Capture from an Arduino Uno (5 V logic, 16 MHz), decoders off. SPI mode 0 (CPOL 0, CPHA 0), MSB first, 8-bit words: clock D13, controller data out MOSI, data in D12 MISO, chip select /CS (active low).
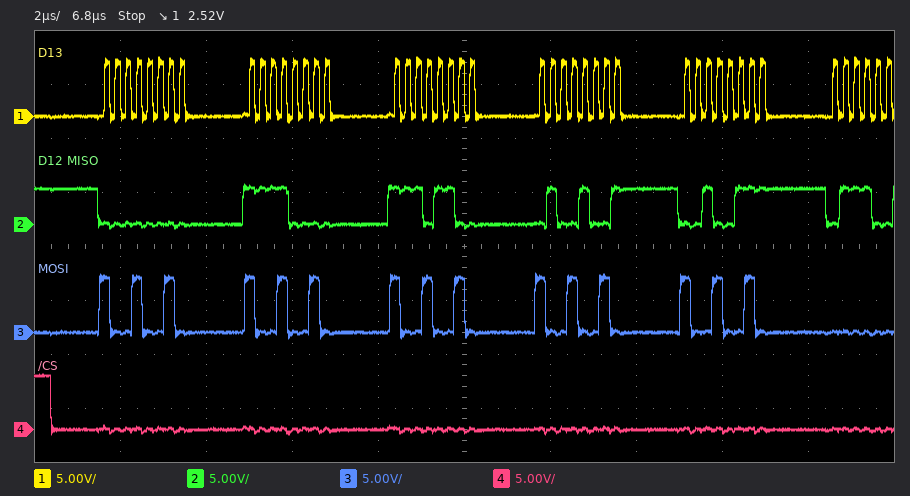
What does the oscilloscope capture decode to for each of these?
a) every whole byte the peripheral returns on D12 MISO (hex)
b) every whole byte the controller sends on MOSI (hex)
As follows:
00 F0 EC 49 27
92 92 92 92 92
